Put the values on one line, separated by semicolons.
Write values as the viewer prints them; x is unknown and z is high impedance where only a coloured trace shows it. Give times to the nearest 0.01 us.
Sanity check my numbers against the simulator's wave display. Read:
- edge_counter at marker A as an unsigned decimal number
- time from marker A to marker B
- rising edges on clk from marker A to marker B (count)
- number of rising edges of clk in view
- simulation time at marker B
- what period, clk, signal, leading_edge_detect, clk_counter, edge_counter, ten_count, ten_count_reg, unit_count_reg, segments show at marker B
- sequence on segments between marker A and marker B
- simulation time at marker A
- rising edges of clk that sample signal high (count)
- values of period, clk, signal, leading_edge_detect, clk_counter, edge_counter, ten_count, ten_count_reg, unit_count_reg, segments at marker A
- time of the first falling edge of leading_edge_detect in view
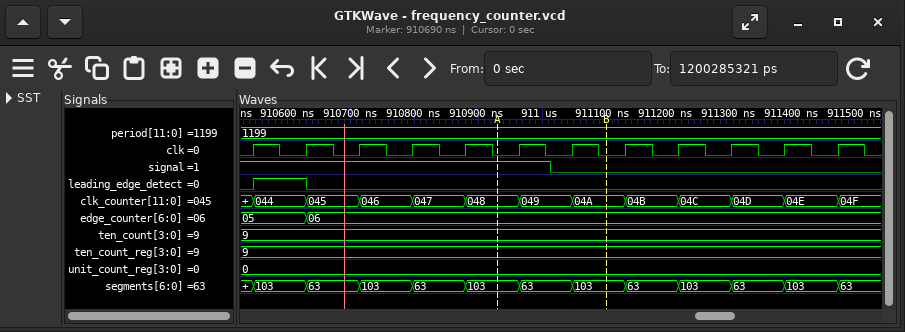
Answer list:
6; 0.17 us; 2; 12; 911.1 us; period=1199, clk=0, signal=0, leading_edge_detect=0, clk_counter=04A, edge_counter=06, ten_count=9, ten_count_reg=9, unit_count_reg=0, segments=103; 103, 63, 103; 910.93 us; 6; period=1199, clk=0, signal=1, leading_edge_detect=0, clk_counter=048, edge_counter=06, ten_count=9, ten_count_reg=9, unit_count_reg=0, segments=103; 910.63 us
